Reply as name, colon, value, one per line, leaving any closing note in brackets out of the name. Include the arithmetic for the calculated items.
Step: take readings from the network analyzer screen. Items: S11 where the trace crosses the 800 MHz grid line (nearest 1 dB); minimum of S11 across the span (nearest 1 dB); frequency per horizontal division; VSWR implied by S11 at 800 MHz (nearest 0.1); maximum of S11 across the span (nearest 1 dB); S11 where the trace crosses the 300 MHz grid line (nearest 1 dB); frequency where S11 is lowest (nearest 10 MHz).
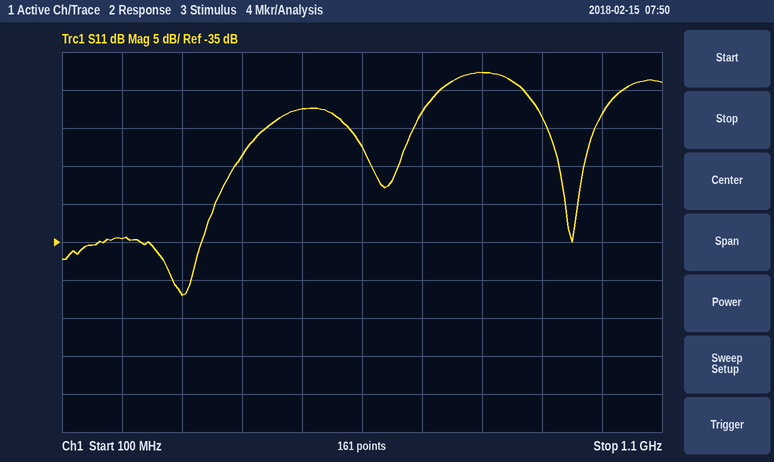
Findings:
S11 where the trace crosses the 800 MHz grid line: -13 dB
minimum of S11 across the span: -42 dB
frequency per horizontal division: 100 MHz
VSWR implied by S11 at 800 MHz: |Γ| = 10^(-13/20) = 0.2239; VSWR = (1 + 0.2239)/(1 − 0.2239) ≈ 1.6
maximum of S11 across the span: -13 dB
S11 where the trace crosses the 300 MHz grid line: -42 dB
frequency where S11 is lowest: 300 MHz
